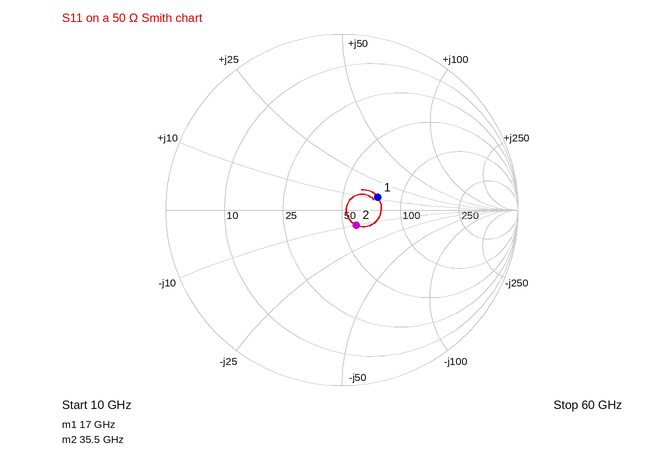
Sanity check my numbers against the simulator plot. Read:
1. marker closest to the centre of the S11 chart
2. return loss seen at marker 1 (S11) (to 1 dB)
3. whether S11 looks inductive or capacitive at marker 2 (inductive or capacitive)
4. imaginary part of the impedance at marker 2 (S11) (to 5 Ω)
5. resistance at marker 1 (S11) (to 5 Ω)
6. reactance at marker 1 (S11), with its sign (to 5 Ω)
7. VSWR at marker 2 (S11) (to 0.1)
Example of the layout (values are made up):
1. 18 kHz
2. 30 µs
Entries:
1. marker 2
2. 13 dB
3. capacitive
4. -10 Ω
5. 75 Ω
6. +10 Ω
7. 1.3
